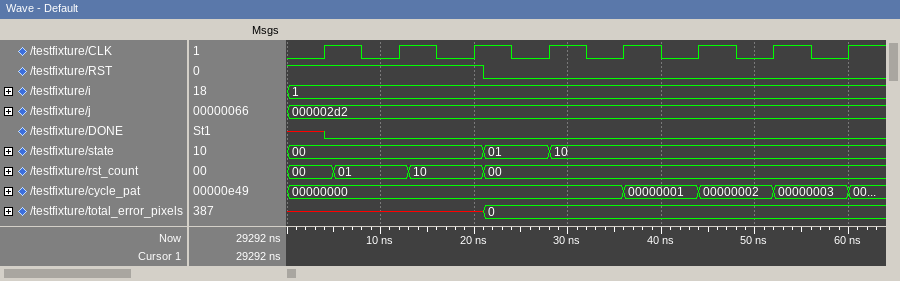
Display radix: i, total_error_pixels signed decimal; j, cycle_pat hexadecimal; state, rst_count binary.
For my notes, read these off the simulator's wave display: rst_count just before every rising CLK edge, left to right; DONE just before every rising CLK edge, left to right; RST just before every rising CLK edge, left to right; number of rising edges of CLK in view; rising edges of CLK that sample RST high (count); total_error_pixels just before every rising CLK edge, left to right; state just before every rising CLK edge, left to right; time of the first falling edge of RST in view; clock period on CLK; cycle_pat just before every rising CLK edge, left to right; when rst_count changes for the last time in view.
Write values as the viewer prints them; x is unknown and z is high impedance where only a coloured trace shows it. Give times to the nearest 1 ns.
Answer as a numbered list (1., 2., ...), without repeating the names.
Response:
1. 00, 01, 10, 00, 00, 00, 00, 00
2. x 0 0 0 0 0 0 0
3. 1 1 1 0 0 0 0 0
4. 8
5. 3
6. x, x, x, 0, 0, 0, 0, 0
7. 00, 00, 00, 01, 10, 10, 10, 10
8. 21 ns
9. 8 ns
10. 00000000, 00000000, 00000000, 00000000, 00000000, 00000001, 00000002, 00000003
11. 21 ns
